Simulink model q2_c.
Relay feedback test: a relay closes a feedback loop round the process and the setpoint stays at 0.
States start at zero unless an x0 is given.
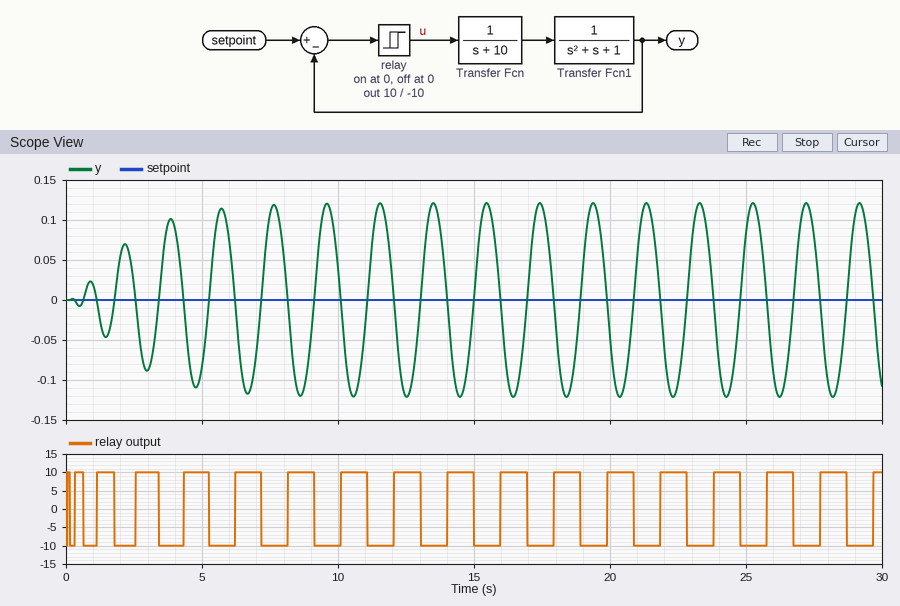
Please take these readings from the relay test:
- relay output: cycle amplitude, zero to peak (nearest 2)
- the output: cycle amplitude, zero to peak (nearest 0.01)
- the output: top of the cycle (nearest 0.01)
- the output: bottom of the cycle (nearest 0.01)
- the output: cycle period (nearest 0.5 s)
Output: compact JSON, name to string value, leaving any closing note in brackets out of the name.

{"relay output: cycle amplitude, zero to peak": "10", "the output: cycle amplitude, zero to peak": "0.12", "the output: top of the cycle": "0.12", "the output: bottom of the cycle": "-0.12", "the output: cycle period": "2.0 s"}
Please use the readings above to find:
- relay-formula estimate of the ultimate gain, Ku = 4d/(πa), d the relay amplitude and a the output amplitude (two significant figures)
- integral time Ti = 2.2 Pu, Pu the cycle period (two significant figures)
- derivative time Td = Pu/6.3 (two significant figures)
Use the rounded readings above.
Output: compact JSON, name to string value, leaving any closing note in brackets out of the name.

{"relay-formula estimate of the ultimate gain, Ku = 4d/(πa), d the relay amplitude and a the output amplitude": "110", "integral time Ti = 2.2 Pu, Pu the cycle period": "4.4 s", "derivative time Td = Pu/6.3": "0.32 s"}
